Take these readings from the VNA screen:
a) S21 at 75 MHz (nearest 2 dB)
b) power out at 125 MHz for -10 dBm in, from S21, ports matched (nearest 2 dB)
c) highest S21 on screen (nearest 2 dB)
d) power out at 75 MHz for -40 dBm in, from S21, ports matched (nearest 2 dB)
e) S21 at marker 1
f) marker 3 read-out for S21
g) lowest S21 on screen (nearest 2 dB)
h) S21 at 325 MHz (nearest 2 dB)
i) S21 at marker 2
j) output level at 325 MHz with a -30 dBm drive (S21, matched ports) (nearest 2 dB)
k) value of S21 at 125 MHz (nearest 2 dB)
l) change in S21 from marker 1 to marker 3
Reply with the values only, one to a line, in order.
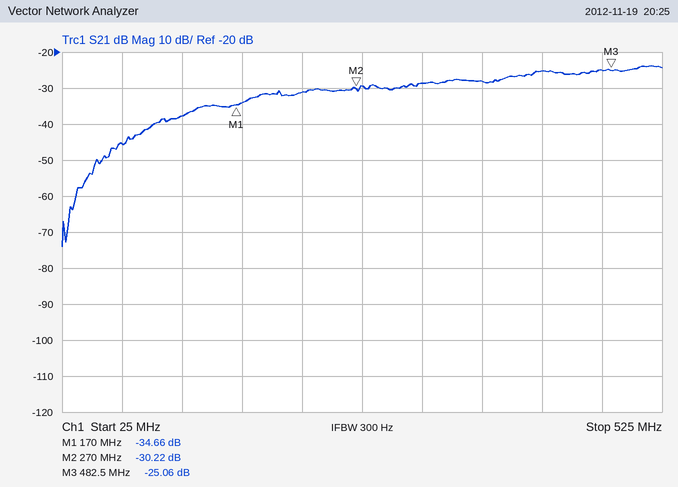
-46 dB
-48 dBm
-24 dB
-86 dBm
-34.66 dB
-25.06 dB
-74 dB
-28 dB
-30.22 dB
-58 dBm
-38 dB
9.60 dB
